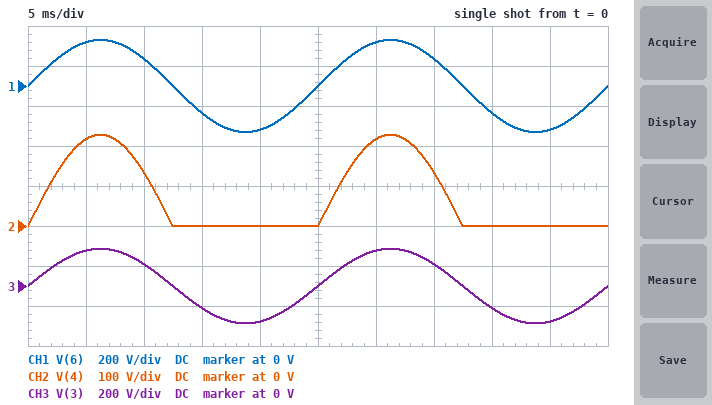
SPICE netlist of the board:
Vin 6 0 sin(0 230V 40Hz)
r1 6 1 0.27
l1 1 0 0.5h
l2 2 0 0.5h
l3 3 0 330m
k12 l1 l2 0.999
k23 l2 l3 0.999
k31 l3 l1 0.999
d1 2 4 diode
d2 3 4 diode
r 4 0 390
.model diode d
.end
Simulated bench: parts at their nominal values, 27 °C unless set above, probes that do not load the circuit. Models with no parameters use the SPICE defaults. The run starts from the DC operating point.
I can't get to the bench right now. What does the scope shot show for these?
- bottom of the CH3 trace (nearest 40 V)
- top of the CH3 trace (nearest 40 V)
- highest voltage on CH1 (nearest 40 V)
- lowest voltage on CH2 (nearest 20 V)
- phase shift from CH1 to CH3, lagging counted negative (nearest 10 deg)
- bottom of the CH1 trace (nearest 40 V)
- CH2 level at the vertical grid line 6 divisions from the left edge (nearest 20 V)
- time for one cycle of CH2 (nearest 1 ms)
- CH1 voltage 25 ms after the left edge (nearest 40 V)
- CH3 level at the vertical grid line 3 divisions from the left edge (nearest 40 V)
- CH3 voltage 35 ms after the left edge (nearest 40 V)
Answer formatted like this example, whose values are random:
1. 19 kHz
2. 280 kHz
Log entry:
1. -200 V
2. 200 V
3. 240 V
4. 0 V
5. 0 deg
6. -240 V
7. 220 V
8. 25 ms
9. 0 V
10. -120 V
11. 120 V
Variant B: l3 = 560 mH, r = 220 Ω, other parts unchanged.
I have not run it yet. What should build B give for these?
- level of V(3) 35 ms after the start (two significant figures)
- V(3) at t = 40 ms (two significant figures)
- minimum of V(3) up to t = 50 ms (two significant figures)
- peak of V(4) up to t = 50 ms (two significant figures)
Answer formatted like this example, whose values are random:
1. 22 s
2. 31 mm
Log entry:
1. 140 V
2. -140 V
3. -240 V
4. 240 V
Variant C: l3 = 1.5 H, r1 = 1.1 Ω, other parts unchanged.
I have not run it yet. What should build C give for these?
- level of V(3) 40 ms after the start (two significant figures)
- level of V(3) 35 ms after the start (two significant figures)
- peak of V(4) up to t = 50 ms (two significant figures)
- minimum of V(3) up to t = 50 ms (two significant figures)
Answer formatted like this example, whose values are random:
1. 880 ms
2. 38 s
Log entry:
1. -240 V
2. 230 V
3. 390 V
4. -400 V
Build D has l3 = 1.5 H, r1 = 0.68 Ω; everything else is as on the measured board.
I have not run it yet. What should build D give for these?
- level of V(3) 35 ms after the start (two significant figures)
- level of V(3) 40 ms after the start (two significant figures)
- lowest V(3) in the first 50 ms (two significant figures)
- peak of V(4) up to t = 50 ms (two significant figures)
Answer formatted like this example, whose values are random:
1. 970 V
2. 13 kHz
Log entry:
1. 230 V
2. -240 V
3. -400 V
4. 390 V
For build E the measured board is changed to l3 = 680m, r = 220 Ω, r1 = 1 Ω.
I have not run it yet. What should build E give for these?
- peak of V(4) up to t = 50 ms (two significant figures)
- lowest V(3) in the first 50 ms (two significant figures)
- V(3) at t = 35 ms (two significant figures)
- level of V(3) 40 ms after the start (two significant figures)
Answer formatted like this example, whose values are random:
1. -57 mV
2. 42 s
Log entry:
1. 260 V
2. -270 V
3. 150 V
4. -160 V
